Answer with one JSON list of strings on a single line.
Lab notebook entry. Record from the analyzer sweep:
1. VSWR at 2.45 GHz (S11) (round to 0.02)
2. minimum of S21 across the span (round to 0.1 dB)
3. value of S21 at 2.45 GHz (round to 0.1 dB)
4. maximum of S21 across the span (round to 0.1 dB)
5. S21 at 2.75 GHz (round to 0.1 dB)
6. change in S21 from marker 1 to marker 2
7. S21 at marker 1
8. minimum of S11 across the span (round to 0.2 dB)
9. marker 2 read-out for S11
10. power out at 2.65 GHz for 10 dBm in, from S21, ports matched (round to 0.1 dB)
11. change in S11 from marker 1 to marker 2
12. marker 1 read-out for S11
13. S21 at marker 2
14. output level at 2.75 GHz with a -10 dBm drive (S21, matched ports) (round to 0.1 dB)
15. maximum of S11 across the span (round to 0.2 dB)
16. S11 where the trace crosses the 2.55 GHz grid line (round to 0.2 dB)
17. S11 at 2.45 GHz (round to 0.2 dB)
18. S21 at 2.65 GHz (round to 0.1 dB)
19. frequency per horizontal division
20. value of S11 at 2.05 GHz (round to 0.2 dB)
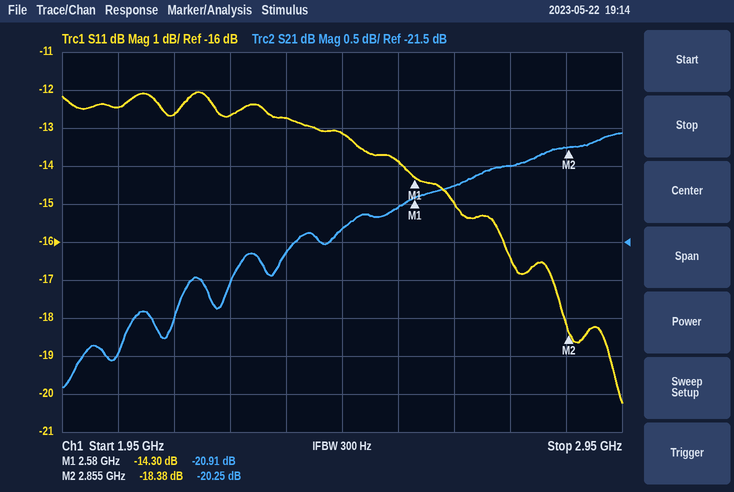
["1.56", "-23.4 dB", "-21.3 dB", "-20.1 dB", "-20.5 dB", "0.66 dB", "-20.91 dB", "-20.2 dB", "-18.38 dB", "-10.8 dBm", "-4.08 dB", "-14.30 dB", "-20.25 dB", "-30.5 dBm", "-12.0 dB", "-13.8 dB", "-13.2 dB", "-20.8 dB", "100 MHz", "-12.4 dB"]
